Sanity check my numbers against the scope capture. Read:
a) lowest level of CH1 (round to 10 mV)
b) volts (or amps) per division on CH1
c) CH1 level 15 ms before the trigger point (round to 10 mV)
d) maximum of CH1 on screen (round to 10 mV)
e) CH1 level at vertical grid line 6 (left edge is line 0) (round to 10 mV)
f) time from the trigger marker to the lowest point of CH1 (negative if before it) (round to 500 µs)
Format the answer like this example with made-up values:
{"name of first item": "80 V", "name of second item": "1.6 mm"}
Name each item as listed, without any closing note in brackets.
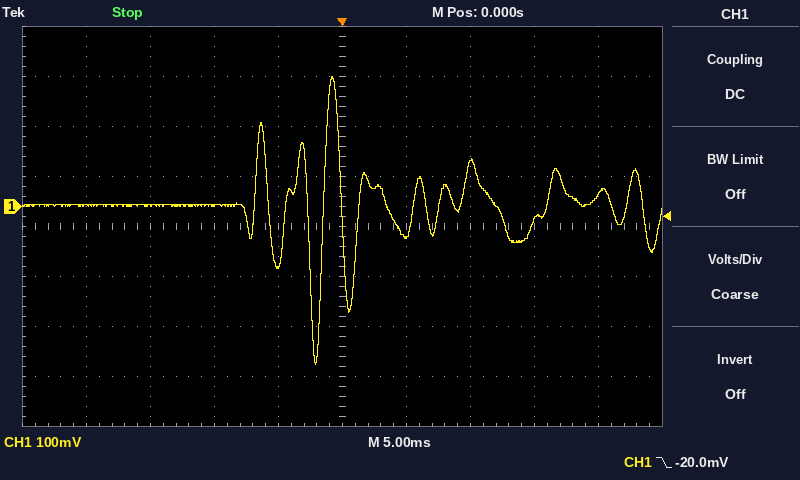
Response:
{"lowest level of CH1": "-320 mV", "volts (or amps) per division on CH1": "100 mV", "CH1 level 15 ms before the trigger point": "0 mV", "maximum of CH1 on screen": "260 mV", "CH1 level at vertical grid line 6 (left edge is line 0)": "-60 mV", "time from the trigger marker to the lowest point of CH1 (negative if before it)": "-2.0 ms"}
